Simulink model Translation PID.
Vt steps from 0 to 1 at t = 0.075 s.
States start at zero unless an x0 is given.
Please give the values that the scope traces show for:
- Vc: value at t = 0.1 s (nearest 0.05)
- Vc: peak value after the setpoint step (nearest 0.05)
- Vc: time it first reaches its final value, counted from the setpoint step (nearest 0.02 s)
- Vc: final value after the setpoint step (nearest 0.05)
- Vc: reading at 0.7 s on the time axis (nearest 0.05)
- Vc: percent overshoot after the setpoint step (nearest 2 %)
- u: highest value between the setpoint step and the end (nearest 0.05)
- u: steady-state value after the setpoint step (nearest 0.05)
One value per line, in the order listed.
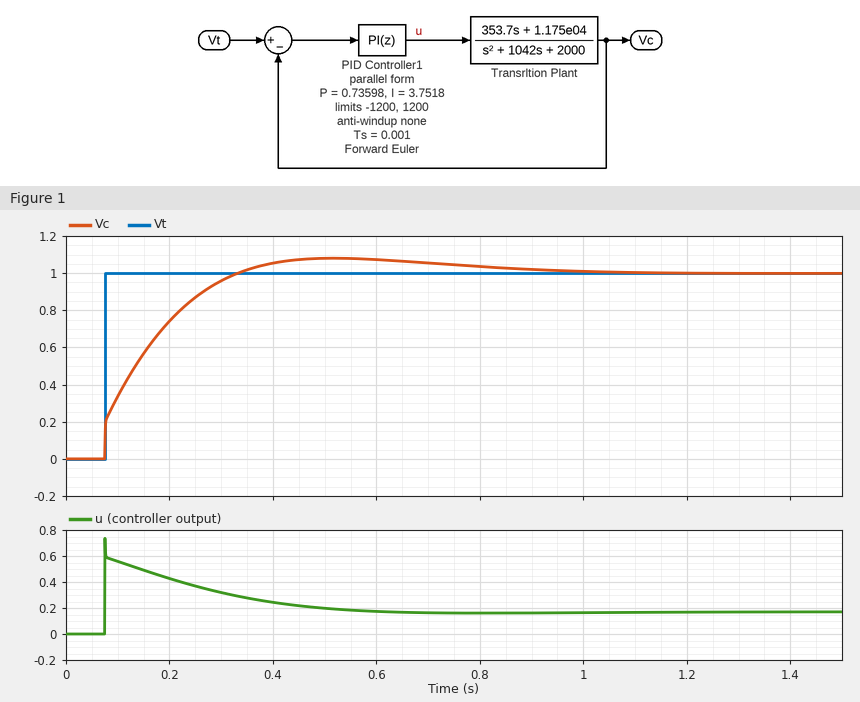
0.35
1.10
0.26 s
1.00
1.05
8 %
0.75
0.15
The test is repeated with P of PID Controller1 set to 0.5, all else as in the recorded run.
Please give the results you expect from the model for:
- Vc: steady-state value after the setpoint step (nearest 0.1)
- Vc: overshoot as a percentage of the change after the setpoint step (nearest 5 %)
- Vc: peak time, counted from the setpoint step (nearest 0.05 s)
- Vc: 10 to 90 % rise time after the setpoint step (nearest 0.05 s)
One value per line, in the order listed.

1.0
15 %
0.45 s
0.20 s
